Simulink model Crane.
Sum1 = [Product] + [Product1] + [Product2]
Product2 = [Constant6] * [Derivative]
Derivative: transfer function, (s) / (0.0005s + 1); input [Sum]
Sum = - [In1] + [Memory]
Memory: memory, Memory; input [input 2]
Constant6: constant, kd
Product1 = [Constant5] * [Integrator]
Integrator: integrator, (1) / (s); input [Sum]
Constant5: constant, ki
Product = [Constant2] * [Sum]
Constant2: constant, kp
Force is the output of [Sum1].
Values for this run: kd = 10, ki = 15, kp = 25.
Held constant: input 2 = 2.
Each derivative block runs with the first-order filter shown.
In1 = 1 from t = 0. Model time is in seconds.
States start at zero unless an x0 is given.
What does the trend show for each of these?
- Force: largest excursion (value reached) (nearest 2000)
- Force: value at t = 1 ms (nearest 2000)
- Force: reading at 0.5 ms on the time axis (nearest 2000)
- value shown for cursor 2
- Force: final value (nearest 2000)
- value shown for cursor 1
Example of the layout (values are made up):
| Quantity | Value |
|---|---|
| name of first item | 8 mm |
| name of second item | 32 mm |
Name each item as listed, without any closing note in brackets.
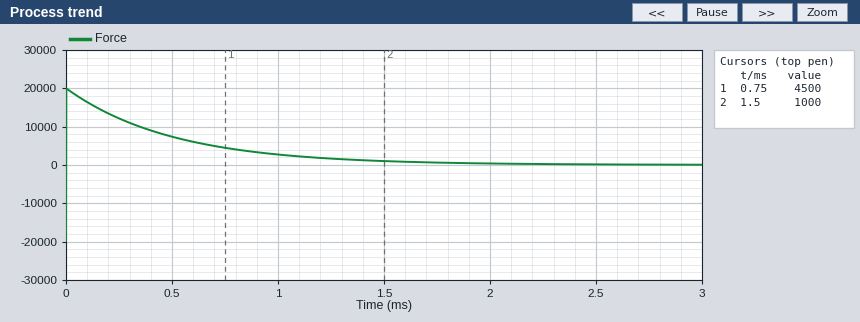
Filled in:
| Quantity | Value |
|---|---|
| Force: largest excursion (value reached) | 20000 |
| Force: value at t = 1 ms | 2000 |
| Force: reading at 0.5 ms on the time axis | 8000 |
| value shown for cursor 2 | 1000 |
| Force: final value | 0 |
| value shown for cursor 1 | 4500 |
